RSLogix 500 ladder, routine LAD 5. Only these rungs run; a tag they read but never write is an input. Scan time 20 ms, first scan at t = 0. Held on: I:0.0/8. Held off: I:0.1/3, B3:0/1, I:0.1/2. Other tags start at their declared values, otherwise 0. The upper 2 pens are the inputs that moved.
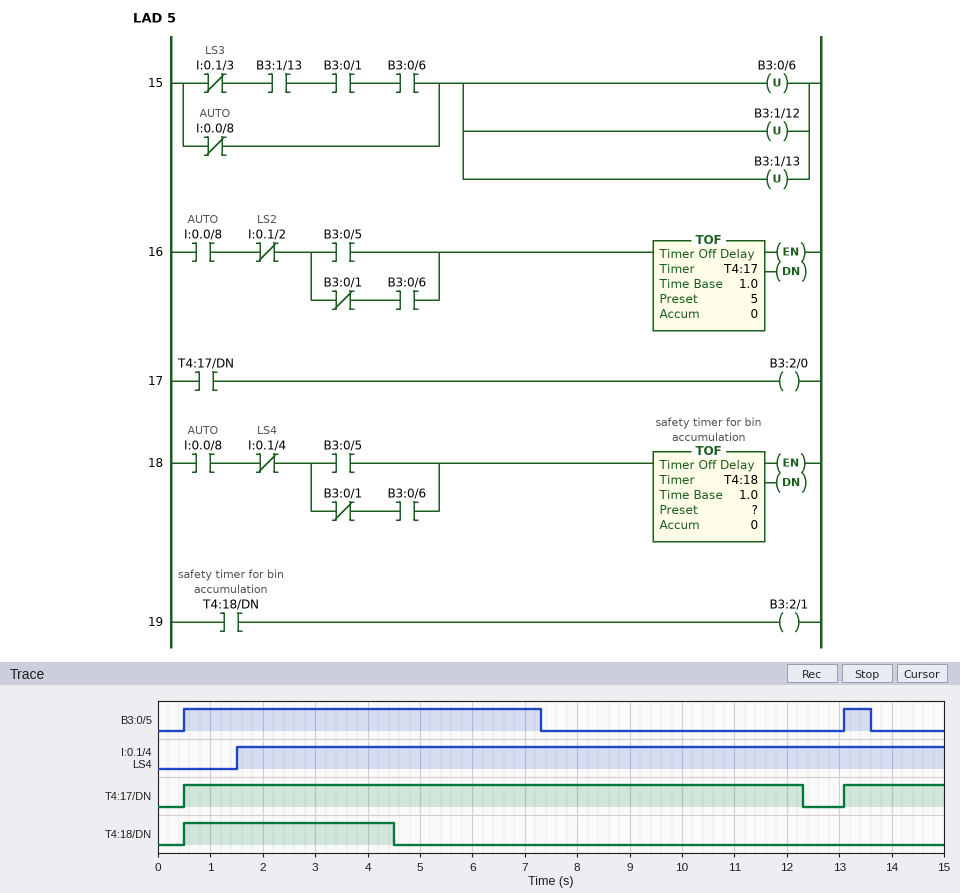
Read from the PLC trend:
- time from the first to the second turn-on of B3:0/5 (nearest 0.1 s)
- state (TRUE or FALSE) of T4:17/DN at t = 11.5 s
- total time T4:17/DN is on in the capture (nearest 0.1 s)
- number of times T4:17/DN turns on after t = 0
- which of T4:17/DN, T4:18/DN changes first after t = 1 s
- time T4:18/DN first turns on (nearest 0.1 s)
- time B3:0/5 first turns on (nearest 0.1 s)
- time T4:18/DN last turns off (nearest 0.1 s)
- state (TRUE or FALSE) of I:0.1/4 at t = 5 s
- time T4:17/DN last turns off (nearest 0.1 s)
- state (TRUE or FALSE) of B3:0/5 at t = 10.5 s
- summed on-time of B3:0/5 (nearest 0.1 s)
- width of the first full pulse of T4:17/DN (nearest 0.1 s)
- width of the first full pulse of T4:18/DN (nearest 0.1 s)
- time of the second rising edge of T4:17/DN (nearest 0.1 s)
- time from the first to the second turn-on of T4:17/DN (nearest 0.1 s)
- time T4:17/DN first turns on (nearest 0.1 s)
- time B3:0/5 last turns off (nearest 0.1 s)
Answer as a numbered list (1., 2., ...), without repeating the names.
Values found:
1. 12.6 s
2. TRUE
3. 13.7 s
4. 2
5. T4:18/DN
6. 0.5 s
7. 0.5 s
8. 4.5 s
9. TRUE
10. 12.3 s
11. FALSE
12. 7.3 s
13. 11.8 s
14. 4.0 s
15. 13.1 s
16. 12.6 s
17. 0.5 s
18. 13.6 s
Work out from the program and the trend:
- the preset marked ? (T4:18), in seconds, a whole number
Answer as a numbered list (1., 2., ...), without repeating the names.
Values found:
1. 3 s
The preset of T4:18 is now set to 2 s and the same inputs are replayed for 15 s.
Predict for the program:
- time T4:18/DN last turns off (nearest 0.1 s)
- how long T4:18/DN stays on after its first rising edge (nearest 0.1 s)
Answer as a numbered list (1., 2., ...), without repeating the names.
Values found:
1. 3.5 s
2. 3.0 s
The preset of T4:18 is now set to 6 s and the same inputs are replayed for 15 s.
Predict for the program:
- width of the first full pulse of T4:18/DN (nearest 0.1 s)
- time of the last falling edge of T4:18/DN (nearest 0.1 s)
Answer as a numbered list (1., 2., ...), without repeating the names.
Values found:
1. 7.0 s
2. 7.5 s
